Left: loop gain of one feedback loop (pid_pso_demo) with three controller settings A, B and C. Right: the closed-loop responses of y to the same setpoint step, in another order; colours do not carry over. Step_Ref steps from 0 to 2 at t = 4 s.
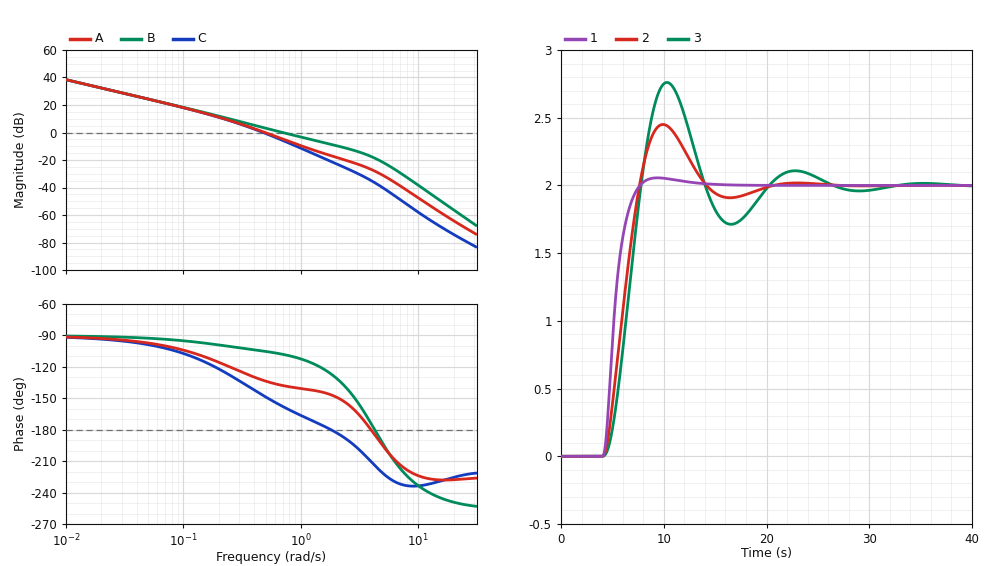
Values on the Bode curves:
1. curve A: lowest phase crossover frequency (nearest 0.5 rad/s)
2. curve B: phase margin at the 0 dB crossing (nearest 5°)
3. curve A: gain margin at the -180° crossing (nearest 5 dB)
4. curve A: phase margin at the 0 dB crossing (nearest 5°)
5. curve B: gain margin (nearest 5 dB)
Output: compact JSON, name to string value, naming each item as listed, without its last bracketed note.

{"curve A: lowest phase crossover frequency": "4.0 rad/s", "curve B: phase margin at the 0 dB crossing": "70°", "curve A: gain margin at the -180° crossing": "25 dB", "curve A: phase margin at the 0 dB crossing": "45°", "curve B: gain margin": "20 dB"}
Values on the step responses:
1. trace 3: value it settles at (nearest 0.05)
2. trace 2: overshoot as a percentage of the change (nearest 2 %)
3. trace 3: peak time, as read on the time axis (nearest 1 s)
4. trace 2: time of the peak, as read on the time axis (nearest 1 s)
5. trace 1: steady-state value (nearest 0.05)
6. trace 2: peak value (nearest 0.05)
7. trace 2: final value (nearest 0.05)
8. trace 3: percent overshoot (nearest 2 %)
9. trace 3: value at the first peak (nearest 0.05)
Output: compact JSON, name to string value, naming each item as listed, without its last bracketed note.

{"trace 3: value it settles at": "2.00", "trace 2: overshoot as a percentage of the change": "22 %", "trace 3: peak time, as read on the time axis": "10 s", "trace 2: time of the peak, as read on the time axis": "10 s", "trace 1: steady-state value": "2.00", "trace 2: peak value": "2.45", "trace 2: final value": "2.00", "trace 3: percent overshoot": "38 %", "trace 3: value at the first peak": "2.75"}
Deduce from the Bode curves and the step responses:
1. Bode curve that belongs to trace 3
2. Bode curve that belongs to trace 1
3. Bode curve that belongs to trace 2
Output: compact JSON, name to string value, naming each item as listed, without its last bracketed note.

{"Bode curve that belongs to trace 3": "C", "Bode curve that belongs to trace 1": "B", "Bode curve that belongs to trace 2": "A"}
